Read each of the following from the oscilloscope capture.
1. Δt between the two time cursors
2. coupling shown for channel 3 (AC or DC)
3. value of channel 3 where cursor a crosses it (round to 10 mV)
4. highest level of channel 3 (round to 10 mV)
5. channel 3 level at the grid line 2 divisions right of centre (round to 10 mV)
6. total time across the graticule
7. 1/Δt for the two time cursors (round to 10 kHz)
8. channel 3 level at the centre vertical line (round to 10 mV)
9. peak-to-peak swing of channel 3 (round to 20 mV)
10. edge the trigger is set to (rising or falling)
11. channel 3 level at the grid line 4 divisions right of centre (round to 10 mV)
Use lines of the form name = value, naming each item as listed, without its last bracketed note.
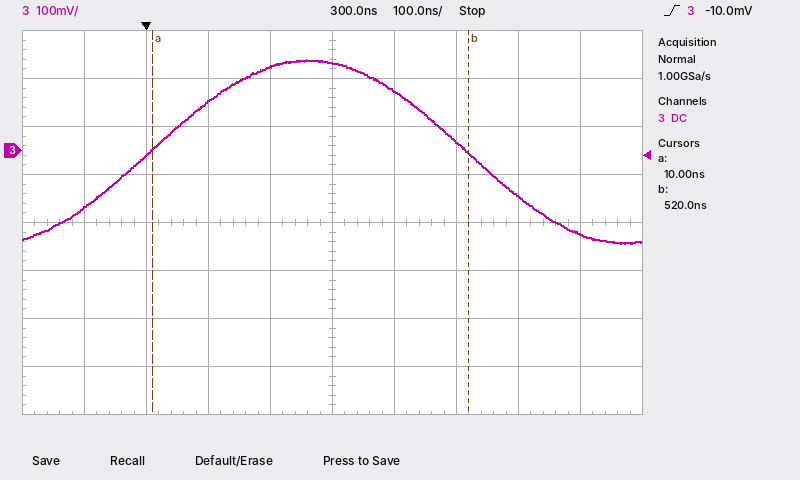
Δt between the two time cursors = 510 ns
coupling shown for channel 3 = DC
value of channel 3 where cursor a crosses it = 0 mV
highest level of channel 3 = 190 mV
channel 3 level at the grid line 2 divisions right of centre = 20 mV
total time across the graticule = 1 µs
1/Δt for the two time cursors = 1.96 MHz
channel 3 level at the centre vertical line = 180 mV
peak-to-peak swing of channel 3 = 380 mV
edge the trigger is set to = rising
channel 3 level at the grid line 4 divisions right of centre = -170 mV
